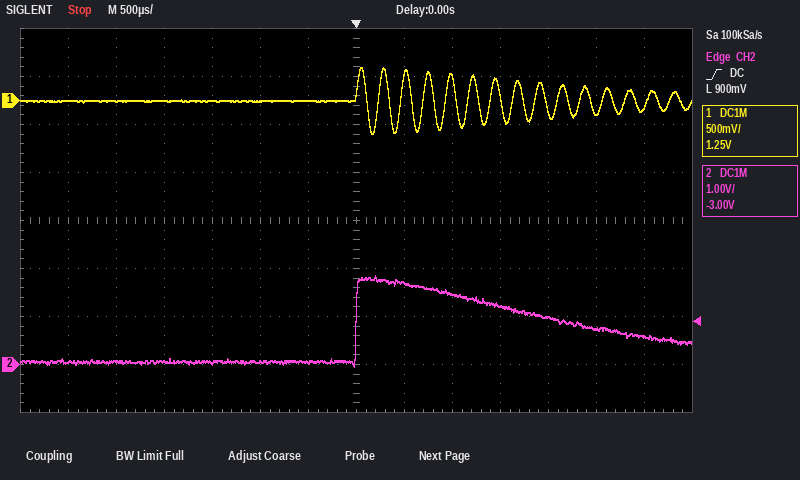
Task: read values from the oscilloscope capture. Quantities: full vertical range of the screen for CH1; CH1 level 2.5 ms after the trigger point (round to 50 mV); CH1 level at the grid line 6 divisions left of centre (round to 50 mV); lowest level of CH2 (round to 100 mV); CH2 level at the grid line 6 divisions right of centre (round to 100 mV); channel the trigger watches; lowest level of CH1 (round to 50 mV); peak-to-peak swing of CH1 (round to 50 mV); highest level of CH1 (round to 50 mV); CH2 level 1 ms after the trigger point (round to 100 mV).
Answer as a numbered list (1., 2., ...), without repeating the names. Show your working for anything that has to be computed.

1. 4 V
2. -150 mV
3. 0 mV
4. 0.0 V
5. 600 mV
6. CH2
7. -350 mV
8. 350 mV − (-350 mV) = 700 mV
9. 350 mV
10. 1.5 V
